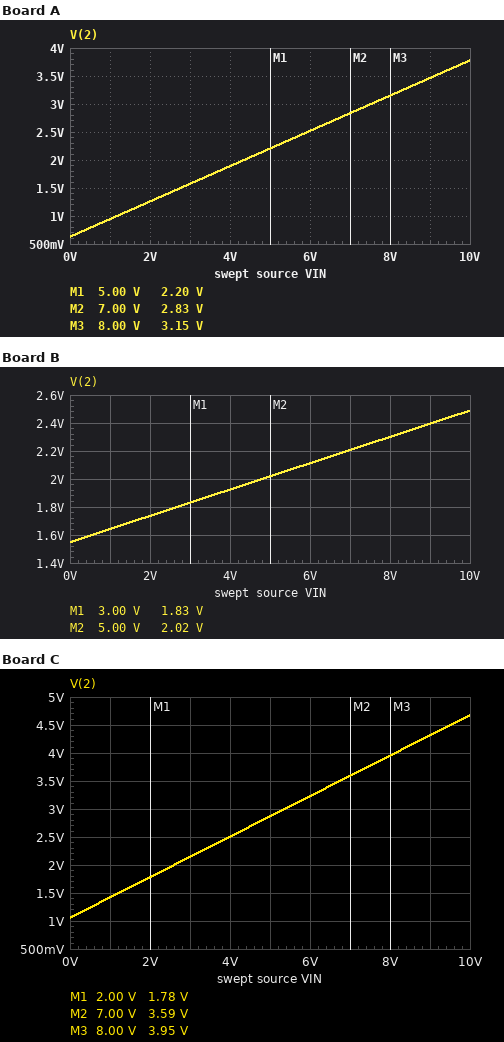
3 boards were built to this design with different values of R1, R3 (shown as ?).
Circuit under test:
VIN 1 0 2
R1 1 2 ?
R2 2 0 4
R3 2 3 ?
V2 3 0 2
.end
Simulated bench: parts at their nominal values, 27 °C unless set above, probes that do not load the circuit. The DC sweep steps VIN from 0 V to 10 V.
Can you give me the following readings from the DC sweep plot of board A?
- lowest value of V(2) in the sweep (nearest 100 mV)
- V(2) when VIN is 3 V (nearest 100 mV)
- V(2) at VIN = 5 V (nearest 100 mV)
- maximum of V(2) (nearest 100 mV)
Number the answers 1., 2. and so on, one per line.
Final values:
1. 600 mV
2. 1.6 V
3. 2.2 V
4. 3.8 V
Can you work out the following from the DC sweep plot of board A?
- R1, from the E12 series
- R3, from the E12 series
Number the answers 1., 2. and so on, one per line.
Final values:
1. 4.7 Ω
2. 4.7 Ω
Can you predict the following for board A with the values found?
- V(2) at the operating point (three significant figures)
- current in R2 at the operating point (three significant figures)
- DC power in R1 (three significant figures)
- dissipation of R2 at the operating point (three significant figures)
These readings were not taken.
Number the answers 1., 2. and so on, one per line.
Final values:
1. 1.26 V
2. 315 mA
3. 117 mW
4. 397 mW
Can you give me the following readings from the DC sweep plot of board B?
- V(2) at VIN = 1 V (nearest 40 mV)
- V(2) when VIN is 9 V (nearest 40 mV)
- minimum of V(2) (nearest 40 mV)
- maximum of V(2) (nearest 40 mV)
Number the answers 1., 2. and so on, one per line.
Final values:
1. 1.64 V
2. 2.40 V
3. 1.56 V
4. 2.48 V
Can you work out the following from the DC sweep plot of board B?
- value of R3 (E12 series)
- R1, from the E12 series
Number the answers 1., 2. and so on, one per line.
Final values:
1. 0.68 Ω
2. 5.6 Ω
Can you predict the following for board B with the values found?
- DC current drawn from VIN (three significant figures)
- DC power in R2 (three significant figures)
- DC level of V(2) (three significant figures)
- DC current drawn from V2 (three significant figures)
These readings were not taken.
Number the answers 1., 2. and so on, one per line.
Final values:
1. 47.0 mA
2. 754 mW
3. 1.74 V
4. 387 mA
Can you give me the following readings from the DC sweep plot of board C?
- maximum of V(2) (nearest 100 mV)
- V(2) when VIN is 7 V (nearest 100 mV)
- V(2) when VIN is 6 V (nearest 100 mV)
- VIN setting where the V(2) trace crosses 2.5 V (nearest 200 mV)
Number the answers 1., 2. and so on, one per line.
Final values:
1. 4.7 V
2. 3.6 V
3. 3.2 V
4. 4.0 V
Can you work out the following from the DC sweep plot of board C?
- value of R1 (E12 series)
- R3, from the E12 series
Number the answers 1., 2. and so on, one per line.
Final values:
1. 1.2 Ω
2. 0.82 Ω
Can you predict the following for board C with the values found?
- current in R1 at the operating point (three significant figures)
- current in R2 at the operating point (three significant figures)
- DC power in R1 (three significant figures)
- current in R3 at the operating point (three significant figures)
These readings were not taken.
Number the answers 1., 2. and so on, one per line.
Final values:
1. 181 mA
2. 446 mA
3. 39.3 mW
4. 265 mA
